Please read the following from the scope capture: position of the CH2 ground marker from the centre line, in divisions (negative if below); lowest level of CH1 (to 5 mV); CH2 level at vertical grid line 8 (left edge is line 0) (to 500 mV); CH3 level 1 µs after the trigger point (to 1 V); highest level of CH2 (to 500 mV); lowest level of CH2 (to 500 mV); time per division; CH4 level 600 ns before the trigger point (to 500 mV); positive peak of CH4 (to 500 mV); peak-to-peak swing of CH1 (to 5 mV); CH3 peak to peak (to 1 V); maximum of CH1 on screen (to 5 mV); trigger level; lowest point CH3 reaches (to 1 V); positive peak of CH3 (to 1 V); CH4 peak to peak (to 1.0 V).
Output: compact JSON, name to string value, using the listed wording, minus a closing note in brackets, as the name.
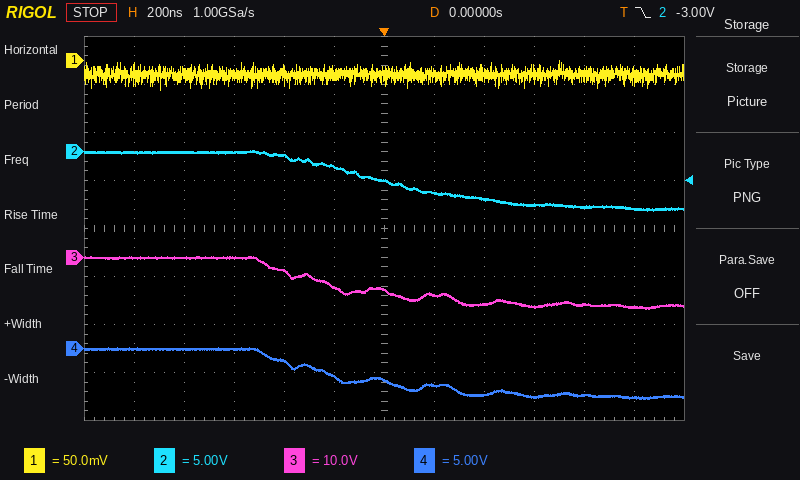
{"position of the CH2 ground marker from the centre line, in divisions": "+1.6 div", "lowest level of CH1": "-30 mV", "CH2 level at vertical grid line 8 (left edge is line 0)": "-5.0 V", "CH3 level 1 µs after the trigger point": "-10 V", "highest level of CH2": "0.0 V", "lowest level of CH2": "-6.0 V", "time per division": "200 ns", "CH4 level 600 ns before the trigger point": "0.0 V", "positive peak of CH4": "0.0 V", "peak-to-peak swing of CH1": "30 mV", "CH3 peak to peak": "11 V", "maximum of CH1 on screen": "0 mV", "trigger level": "-3.00 V", "lowest point CH3 reaches": "-11 V", "positive peak of CH3": "0 V", "CH4 peak to peak": "5.0 V"}
